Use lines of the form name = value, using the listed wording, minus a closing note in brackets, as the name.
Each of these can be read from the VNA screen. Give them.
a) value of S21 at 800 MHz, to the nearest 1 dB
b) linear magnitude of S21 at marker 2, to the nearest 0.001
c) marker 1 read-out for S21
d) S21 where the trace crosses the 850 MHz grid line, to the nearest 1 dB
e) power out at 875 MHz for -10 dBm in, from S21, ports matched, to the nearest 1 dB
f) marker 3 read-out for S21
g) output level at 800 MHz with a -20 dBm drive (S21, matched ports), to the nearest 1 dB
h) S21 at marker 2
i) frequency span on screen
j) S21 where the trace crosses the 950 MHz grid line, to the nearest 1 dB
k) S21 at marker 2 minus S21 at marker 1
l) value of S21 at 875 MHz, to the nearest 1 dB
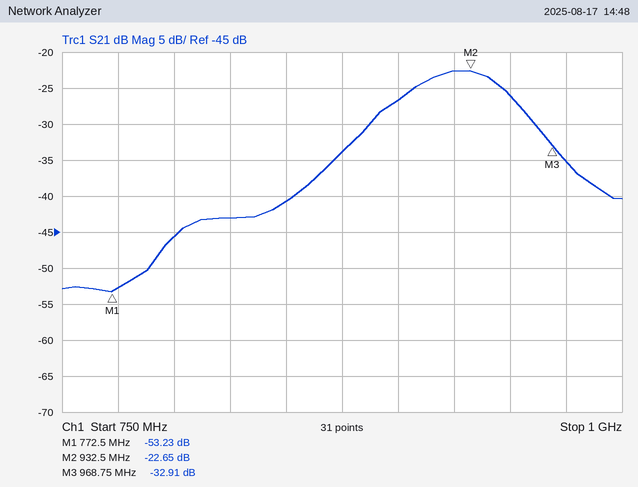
value of S21 at 800 MHz, to the nearest 1 dB = -46 dB
linear magnitude of S21 at marker 2, to the nearest 0.001 = 0.074
marker 1 read-out for S21 = -53.23 dB
S21 where the trace crosses the 850 MHz grid line, to the nearest 1 dB = -41 dB
power out at 875 MHz for -10 dBm in, from S21, ports matched, to the nearest 1 dB = -44 dBm
marker 3 read-out for S21 = -32.91 dB
output level at 800 MHz with a -20 dBm drive (S21, matched ports), to the nearest 1 dB = -66 dBm
S21 at marker 2 = -22.65 dB
frequency span on screen = 250 MHz
S21 where the trace crosses the 950 MHz grid line, to the nearest 1 dB = -26 dB
S21 at marker 2 minus S21 at marker 1 = 30.58 dB
value of S21 at 875 MHz, to the nearest 1 dB = -34 dB
